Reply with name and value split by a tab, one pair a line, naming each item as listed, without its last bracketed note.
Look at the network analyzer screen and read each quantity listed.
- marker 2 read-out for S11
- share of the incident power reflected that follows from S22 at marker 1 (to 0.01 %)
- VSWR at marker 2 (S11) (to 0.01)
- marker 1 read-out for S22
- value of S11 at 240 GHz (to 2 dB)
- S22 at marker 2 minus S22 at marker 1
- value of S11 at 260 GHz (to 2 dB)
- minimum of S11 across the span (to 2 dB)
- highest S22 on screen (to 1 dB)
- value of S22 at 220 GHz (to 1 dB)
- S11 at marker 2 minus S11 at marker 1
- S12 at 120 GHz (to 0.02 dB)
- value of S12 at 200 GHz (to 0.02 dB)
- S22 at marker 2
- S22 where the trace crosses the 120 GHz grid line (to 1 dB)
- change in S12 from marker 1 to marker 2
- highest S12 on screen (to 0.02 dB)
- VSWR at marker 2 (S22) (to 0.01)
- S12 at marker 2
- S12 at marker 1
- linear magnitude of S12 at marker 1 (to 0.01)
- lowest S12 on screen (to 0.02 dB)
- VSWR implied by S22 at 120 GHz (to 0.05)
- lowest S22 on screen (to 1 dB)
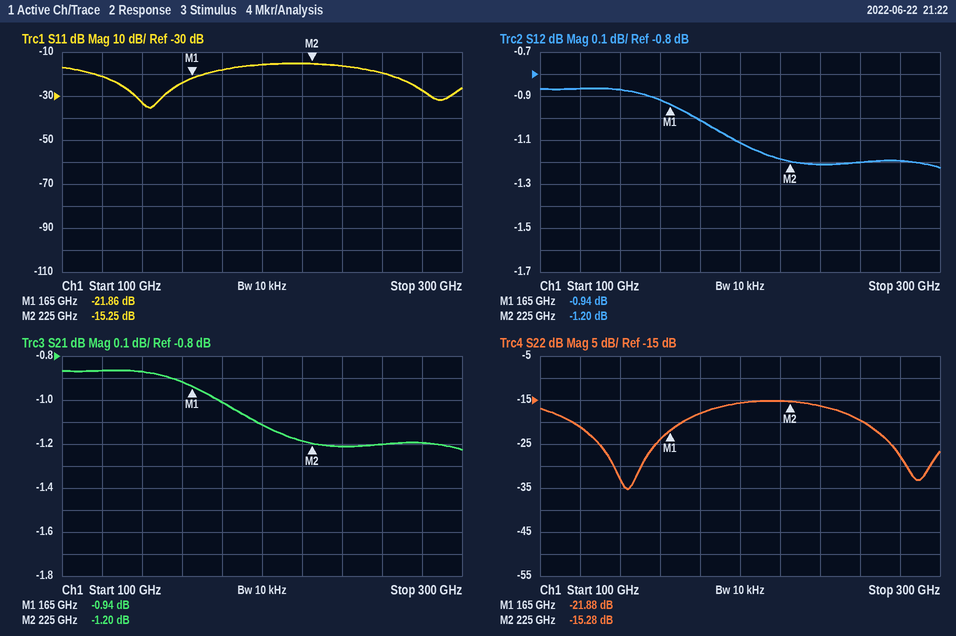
marker 2 read-out for S11	-15.25 dB
share of the incident power reflected that follows from S22 at marker 1	0.65 %
VSWR at marker 2 (S11)	1.42
marker 1 read-out for S22	-21.88 dB
value of S11 at 240 GHz	-16 dB
S22 at marker 2 minus S22 at marker 1	6.60 dB
value of S11 at 260 GHz	-20 dB
minimum of S11 across the span	-36 dB
highest S22 on screen	-15 dB
value of S22 at 220 GHz	-15 dB
S11 at marker 2 minus S11 at marker 1	6.61 dB
S12 at 120 GHz	-0.86 dB
value of S12 at 200 GHz	-1.12 dB
S22 at marker 2	-15.28 dB
S22 where the trace crosses the 120 GHz grid line	-21 dB
change in S12 from marker 1 to marker 2	-0.26 dB
highest S12 on screen	-0.86 dB
VSWR at marker 2 (S22)	1.42
S12 at marker 2	-1.20 dB
S12 at marker 1	-0.94 dB
linear magnitude of S12 at marker 1	0.90
lowest S12 on screen	-1.22 dB
VSWR implied by S22 at 120 GHz	1.20
lowest S22 on screen	-35 dB
